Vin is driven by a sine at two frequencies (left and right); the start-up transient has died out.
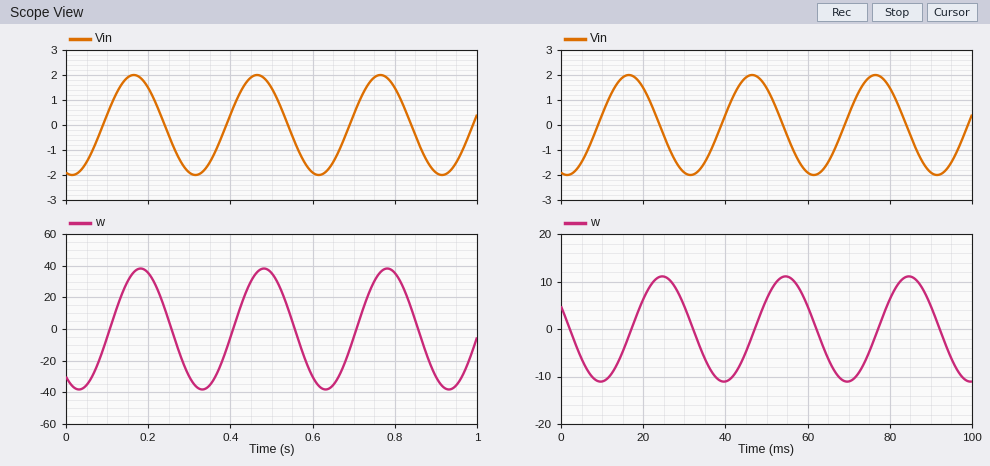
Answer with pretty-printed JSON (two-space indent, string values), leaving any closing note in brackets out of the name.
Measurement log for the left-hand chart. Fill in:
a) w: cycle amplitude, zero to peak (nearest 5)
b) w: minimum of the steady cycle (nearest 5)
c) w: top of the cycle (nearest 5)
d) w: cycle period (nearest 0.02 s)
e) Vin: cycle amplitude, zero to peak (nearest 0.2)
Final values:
{
  "w: cycle amplitude, zero to peak": "40",
  "w: minimum of the steady cycle": "-40",
  "w: top of the cycle": "40",
  "w: cycle period": "0.30 s",
  "Vin: cycle amplitude, zero to peak": "2.0"
}
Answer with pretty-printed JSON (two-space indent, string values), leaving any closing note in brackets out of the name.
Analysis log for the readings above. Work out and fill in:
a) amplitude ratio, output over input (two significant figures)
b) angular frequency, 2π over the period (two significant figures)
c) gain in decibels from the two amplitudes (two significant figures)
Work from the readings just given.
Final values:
{
  "amplitude ratio, output over input": "20",
  "angular frequency, 2π over the period": "21 rad/s",
  "gain in decibels from the two amplitudes": "26 dB"
}
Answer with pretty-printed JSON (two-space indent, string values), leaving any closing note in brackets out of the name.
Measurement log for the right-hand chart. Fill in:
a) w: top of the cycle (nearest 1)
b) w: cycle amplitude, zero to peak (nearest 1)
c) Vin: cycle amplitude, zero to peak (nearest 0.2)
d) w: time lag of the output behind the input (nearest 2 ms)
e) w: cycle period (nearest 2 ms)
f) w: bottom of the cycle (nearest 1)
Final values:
{
  "w: top of the cycle": "11",
  "w: cycle amplitude, zero to peak": "11",
  "Vin: cycle amplitude, zero to peak": "2.0",
  "w: time lag of the output behind the input": "8 ms",
  "w: cycle period": "30 ms",
  "w: bottom of the cycle": "-11"
}
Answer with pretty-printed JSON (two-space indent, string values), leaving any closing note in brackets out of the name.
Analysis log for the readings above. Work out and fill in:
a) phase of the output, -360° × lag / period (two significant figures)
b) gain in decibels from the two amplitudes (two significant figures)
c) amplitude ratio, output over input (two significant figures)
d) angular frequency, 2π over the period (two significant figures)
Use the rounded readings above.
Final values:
{
  "phase of the output, -360° × lag / period": "-96°",
  "gain in decibels from the two amplitudes": "15 dB",
  "amplitude ratio, output over input": "5.5",
  "angular frequency, 2π over the period": "0.21 rad/ms"
}
